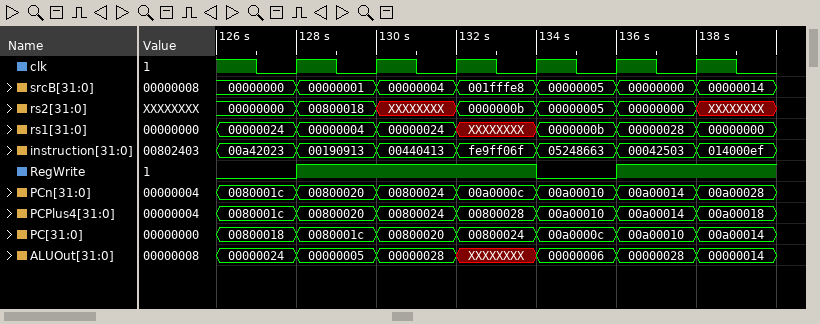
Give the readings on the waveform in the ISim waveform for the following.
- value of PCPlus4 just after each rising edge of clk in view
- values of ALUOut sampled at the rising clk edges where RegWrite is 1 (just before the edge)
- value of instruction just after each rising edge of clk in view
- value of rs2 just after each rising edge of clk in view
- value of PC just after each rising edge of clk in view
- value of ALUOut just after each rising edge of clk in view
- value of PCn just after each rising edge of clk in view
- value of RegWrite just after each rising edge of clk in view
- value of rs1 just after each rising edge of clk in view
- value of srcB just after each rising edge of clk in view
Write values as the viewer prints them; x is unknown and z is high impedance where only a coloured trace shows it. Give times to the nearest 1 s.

00800020, 00800024, 00800028, 00a00010, 00a00014, 00a00018
00000005, 00000028, XXXXXXXX, 00000028
00190913, 00440413, fe9ff06f, 05248663, 00042503, 014000ef
00800018, XXXXXXXX, 0000000b, 00000005, 00000000, XXXXXXXX
0080001c, 00800020, 00800024, 00a0000c, 00a00010, 00a00014
00000005, 00000028, XXXXXXXX, 00000006, 00000028, 00000014
00800020, 00800024, 00a0000c, 00a00010, 00a00014, 00a00028
1 1 1 0 1 1
00000004, 00000024, XXXXXXXX, 0000000b, 00000028, 00000000
00000001, 00000004, 001fffe8, 00000005, 00000000, 00000014
